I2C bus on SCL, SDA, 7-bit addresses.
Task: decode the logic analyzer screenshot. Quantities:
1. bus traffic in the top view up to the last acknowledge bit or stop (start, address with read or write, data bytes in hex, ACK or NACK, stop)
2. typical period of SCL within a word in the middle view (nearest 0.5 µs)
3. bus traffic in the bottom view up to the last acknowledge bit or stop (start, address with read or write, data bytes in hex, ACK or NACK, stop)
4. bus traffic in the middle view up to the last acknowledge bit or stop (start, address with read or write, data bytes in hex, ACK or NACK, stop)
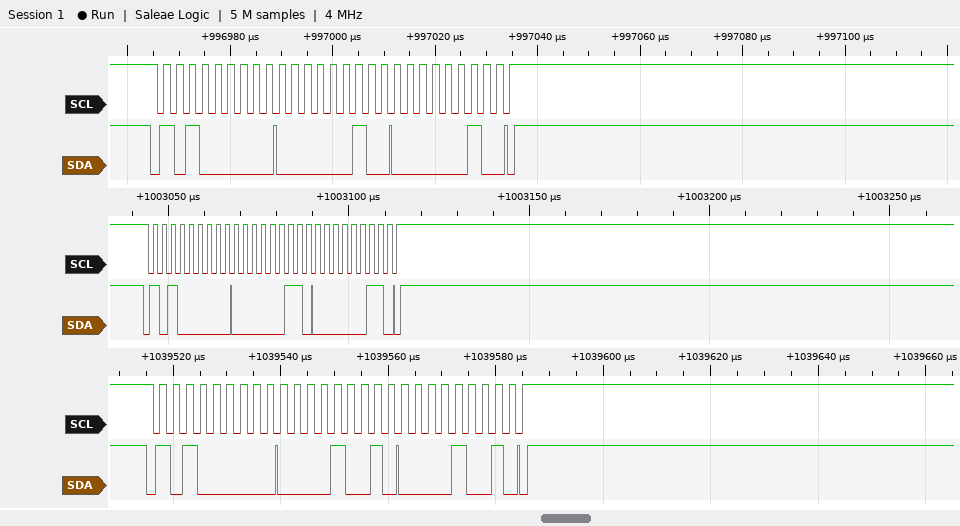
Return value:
start, address 50 write ACK, 02 ACK, 02 ACK, stop
2.5 µs
start, address 50 write ACK, 09 ACK, 09 ACK, stop
start, address 50 write ACK, 03 ACK, 03 ACK, stop
